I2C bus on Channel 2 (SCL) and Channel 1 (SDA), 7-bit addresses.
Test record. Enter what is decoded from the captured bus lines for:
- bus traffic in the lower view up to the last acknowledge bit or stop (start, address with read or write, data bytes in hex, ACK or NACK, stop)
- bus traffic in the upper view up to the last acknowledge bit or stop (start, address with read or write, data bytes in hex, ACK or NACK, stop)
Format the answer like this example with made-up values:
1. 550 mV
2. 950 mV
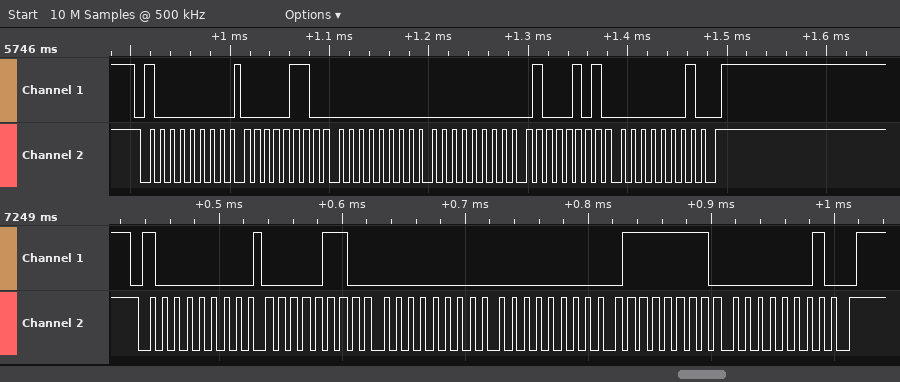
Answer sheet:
1. start, address 40 write ACK, 06 ACK, 00 ACK, 00 ACK, 7F ACK, 01 ACK, stop
2. start, address 40 write ACK, 06 ACK, 00 ACK, 00 ACK, 45 ACK, 01 ACK, stop
